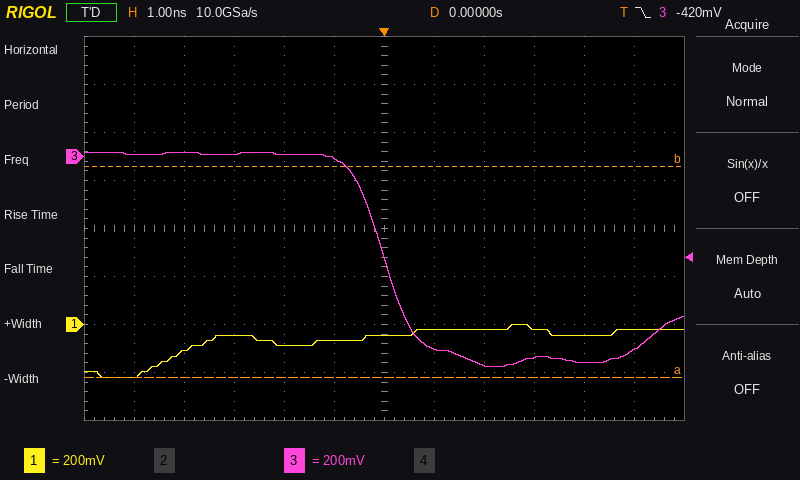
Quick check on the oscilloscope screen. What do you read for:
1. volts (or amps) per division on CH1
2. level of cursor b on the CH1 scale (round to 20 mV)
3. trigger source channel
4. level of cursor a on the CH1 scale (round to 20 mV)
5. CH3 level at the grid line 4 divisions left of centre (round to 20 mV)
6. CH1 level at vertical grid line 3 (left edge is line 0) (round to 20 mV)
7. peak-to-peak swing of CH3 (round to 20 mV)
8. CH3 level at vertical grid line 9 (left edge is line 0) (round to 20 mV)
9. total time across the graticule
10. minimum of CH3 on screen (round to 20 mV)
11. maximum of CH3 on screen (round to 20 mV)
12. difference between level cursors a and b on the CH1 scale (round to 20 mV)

200 mV
660 mV
CH3
-220 mV
20 mV
-40 mV
900 mV
-840 mV
12 ns
-880 mV
20 mV
880 mV
